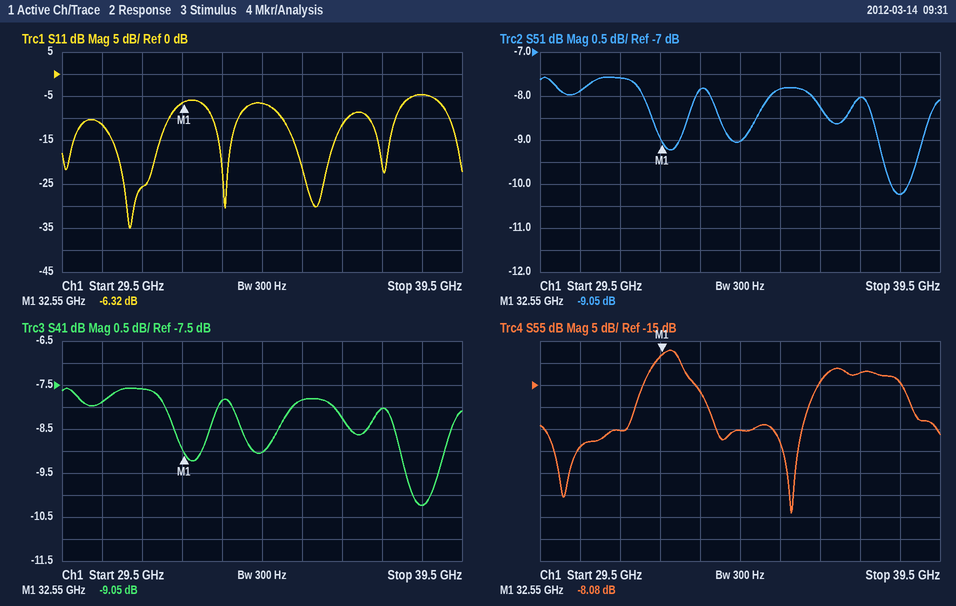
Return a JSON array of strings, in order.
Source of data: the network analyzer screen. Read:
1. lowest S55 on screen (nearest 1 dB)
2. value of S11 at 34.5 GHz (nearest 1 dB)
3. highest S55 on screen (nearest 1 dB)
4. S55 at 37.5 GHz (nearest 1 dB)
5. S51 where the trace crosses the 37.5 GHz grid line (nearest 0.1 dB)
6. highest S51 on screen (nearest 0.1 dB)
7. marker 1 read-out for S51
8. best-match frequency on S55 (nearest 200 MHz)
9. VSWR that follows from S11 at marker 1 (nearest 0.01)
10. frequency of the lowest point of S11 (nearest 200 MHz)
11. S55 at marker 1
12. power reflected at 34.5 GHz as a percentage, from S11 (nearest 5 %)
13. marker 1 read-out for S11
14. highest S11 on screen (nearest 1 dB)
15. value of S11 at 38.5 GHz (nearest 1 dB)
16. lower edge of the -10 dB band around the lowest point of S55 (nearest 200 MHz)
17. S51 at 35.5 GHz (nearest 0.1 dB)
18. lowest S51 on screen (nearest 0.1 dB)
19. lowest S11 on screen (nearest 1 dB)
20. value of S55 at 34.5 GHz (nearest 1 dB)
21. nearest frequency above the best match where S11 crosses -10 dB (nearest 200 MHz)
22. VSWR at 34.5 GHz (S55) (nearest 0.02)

["-44 dB", "-7 dB", "-7 dB", "-12 dB", "-8.0 dB", "-7.6 dB", "-9.05 dB", "35.8 GHz", "2.87", "31.2 GHz", "-8.08 dB", "20 %", "-6.32 dB", "-5 dB", "-5 dB", "33.0 GHz", "-7.8 dB", "-10.2 dB", "-35 dB", "-25 dB", "32.2 GHz", "1.12"]
